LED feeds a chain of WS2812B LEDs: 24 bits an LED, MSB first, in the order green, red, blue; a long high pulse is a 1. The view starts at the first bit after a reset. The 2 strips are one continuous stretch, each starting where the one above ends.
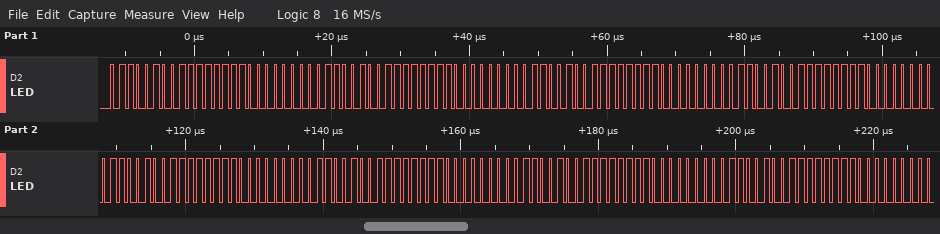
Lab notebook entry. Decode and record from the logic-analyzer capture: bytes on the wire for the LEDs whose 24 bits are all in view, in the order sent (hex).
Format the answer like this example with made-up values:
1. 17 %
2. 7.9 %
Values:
1. 64 FF 00 64 FF 00 64 FF 00 64 FF 00 64 FF 00 64 FF 00 64 FF 00 64 FF 00
